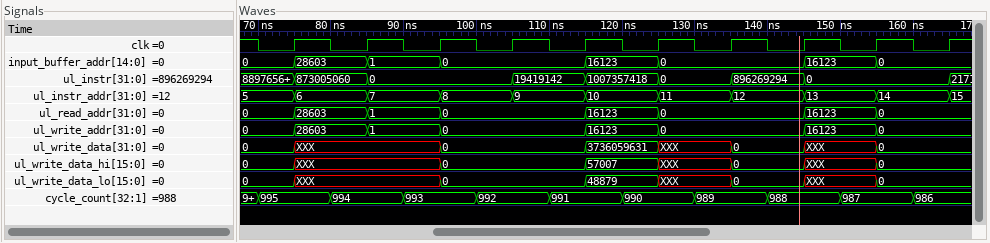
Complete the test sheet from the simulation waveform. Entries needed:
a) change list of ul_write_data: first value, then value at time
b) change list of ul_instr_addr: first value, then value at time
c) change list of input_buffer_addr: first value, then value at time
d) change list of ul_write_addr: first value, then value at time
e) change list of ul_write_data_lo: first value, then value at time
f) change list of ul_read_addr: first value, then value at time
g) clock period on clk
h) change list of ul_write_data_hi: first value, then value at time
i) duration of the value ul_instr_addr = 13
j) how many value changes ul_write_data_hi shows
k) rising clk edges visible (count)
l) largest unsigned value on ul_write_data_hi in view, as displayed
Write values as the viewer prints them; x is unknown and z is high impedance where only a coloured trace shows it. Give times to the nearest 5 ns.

0, XXX at 75 ns, 0 at 95 ns, 3736059631 at 115 ns, XXX at 125 ns, 0 at 135 ns, XXX at 145 ns, 0 at 155 ns
5, 6 at 75 ns, 7 at 85 ns, 8 at 95 ns, 9 at 105 ns, 10 at 115 ns, 11 at 125 ns, 12 at 135 ns, 13 at 145 ns, 14 at 155 ns, 15 at 165 ns
0, 28603 at 75 ns, 1 at 85 ns, 0 at 95 ns, 16123 at 115 ns, 0 at 125 ns, 16123 at 145 ns, 0 at 155 ns
0, 28603 at 75 ns, 1 at 85 ns, 0 at 95 ns, 16123 at 115 ns, 0 at 125 ns, 16123 at 145 ns, 0 at 155 ns
0, XXX at 75 ns, 0 at 95 ns, 48879 at 115 ns, XXX at 125 ns, 0 at 135 ns, XXX at 145 ns, 0 at 155 ns
0, 28603 at 75 ns, 1 at 85 ns, 0 at 95 ns, 16123 at 115 ns, 0 at 125 ns, 16123 at 145 ns, 0 at 155 ns
10 ns
0, XXX at 75 ns, 0 at 95 ns, 57007 at 115 ns, XXX at 125 ns, 0 at 135 ns, XXX at 145 ns, 0 at 155 ns
10 ns
7
10
57007
